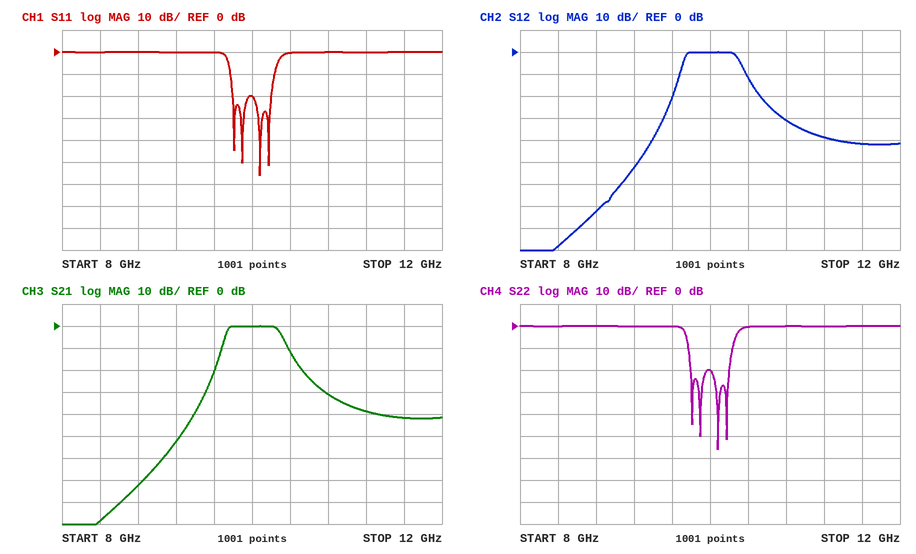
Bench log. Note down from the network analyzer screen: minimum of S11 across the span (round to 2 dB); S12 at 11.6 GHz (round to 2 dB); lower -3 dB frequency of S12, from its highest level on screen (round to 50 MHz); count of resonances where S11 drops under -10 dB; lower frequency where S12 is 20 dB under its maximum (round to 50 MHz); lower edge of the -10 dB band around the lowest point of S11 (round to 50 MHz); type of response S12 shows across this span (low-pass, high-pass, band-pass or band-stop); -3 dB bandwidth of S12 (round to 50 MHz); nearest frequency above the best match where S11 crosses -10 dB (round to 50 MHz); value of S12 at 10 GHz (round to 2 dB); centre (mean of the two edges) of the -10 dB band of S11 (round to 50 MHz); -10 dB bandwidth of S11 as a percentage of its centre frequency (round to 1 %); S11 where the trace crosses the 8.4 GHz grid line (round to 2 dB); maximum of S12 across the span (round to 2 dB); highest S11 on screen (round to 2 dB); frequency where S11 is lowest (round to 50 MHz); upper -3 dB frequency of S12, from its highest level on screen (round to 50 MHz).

-56 dB
-42 dB
9.75 GHz
4
9.60 GHz
9.75 GHz
band-pass
550 MHz
10.25 GHz
0 dB
10.00 GHz
5 %
0 dB
0 dB
0 dB
10.10 GHz
10.30 GHz
